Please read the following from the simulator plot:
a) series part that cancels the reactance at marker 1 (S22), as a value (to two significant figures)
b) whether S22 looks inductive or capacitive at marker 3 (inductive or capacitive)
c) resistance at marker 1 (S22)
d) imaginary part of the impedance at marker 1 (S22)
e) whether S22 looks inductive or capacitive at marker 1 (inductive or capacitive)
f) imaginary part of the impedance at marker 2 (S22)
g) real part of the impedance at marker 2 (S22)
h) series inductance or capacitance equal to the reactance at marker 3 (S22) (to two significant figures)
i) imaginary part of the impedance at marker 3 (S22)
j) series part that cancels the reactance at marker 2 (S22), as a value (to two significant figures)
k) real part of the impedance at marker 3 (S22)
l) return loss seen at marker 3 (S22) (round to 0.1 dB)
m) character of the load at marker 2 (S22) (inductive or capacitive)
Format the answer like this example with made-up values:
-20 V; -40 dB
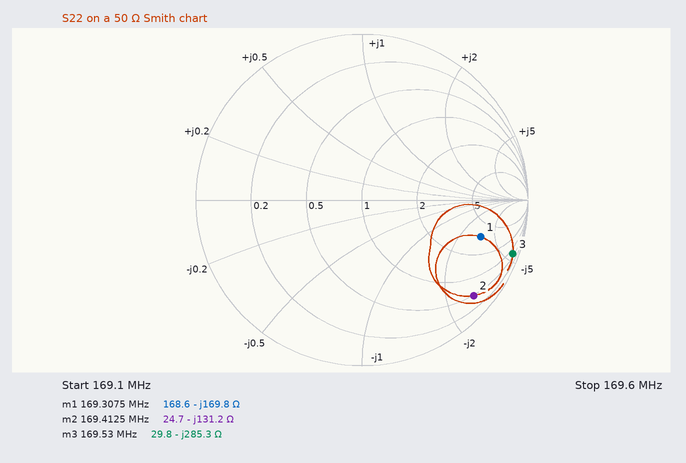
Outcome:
160 nH; capacitive; 168.6 Ω; -169.8 Ω; capacitive; -131.2 Ω; 24.7 Ω; 3.3 pF; -285.3 Ω; 120 nH; 29.8 Ω; 0.3 dB; capacitive
